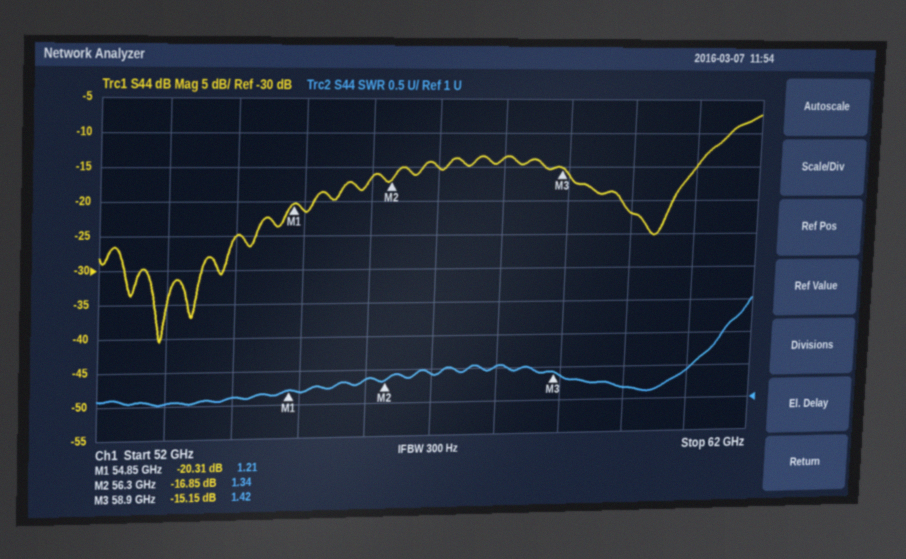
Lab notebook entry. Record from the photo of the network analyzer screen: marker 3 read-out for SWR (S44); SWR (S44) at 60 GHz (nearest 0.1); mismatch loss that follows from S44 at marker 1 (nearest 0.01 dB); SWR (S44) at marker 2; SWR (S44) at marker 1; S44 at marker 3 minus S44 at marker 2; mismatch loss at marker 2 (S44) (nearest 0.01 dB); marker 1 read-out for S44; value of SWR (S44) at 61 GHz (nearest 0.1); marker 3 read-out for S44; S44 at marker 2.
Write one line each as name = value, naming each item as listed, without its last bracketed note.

marker 3 read-out for SWR = 1.42
SWR (S44) at 60 GHz = 1.2
mismatch loss that follows from S44 at marker 1 = 0.04 dB
SWR (S44) at marker 2 = 1.34
SWR (S44) at marker 1 = 1.21
S44 at marker 3 minus S44 at marker 2 = 1.70 dB
mismatch loss at marker 2 (S44) = 0.09 dB
marker 1 read-out for S44 = -20.31 dB
value of SWR (S44) at 61 GHz = 1.4
marker 3 read-out for S44 = -15.15 dB
S44 at marker 2 = -16.85 dB
